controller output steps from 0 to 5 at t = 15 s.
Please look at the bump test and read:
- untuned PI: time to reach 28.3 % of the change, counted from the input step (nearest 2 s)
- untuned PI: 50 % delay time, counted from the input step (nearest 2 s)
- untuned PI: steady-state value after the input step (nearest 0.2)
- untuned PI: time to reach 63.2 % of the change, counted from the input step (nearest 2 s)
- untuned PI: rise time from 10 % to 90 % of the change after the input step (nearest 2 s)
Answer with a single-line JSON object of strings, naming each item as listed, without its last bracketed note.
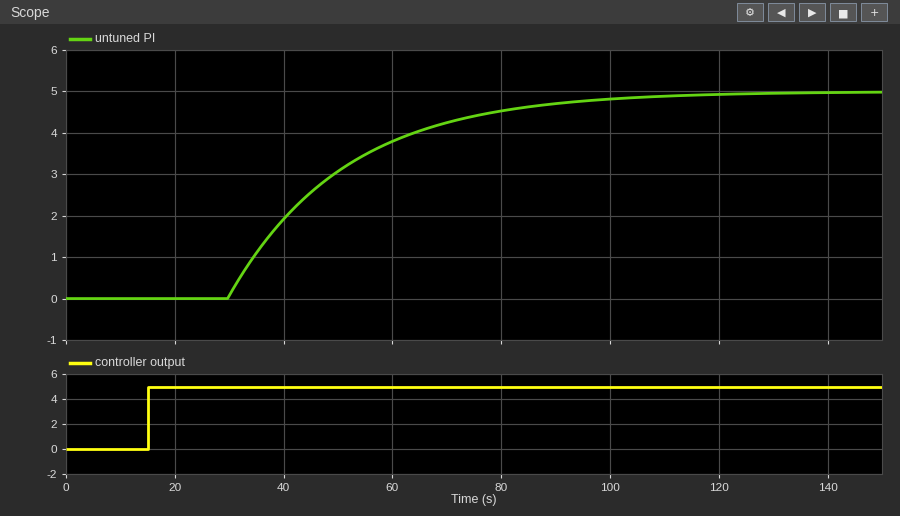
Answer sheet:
{"untuned PI: time to reach 28.3 % of the change, counted from the input step": "22 s", "untuned PI: 50 % delay time, counted from the input step": "30 s", "untuned PI: steady-state value after the input step": "5.0", "untuned PI: time to reach 63.2 % of the change, counted from the input step": "36 s", "untuned PI: rise time from 10 % to 90 % of the change after the input step": "46 s"}
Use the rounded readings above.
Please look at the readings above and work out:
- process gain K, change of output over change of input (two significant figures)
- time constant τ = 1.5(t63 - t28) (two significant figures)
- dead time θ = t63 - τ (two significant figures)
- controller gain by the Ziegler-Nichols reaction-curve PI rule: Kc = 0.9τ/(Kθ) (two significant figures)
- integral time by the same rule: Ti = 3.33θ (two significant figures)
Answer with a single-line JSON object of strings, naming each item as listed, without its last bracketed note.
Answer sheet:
{"process gain K, change of output over change of input": "1.0", "time constant τ = 1.5(t63 - t28)": "21 s", "dead time θ = t63 - τ": "15 s", "controller gain by the Ziegler-Nichols reaction-curve PI rule: Kc = 0.9τ/(Kθ)": "1.3", "integral time by the same rule: Ti = 3.33θ": "50 s"}
